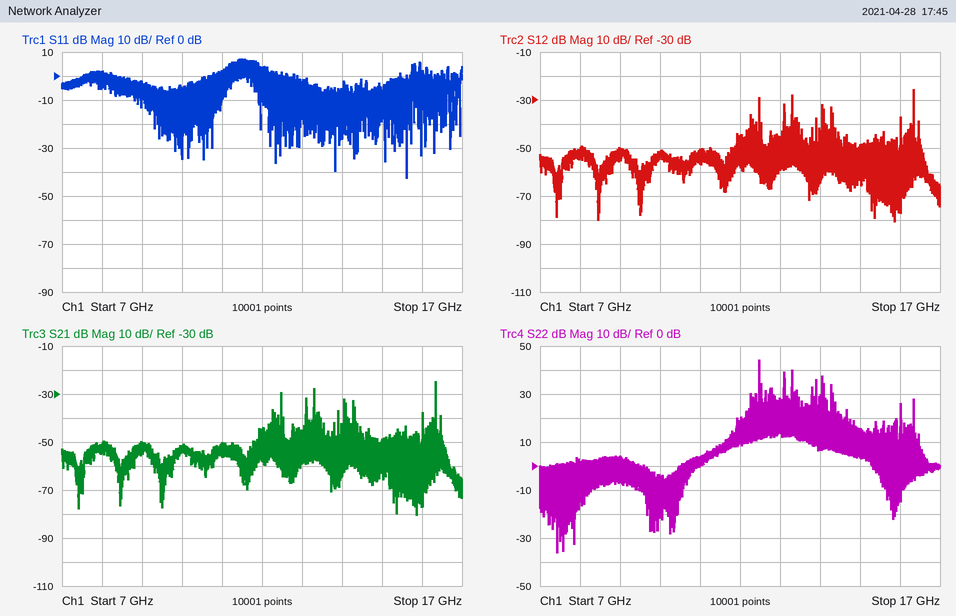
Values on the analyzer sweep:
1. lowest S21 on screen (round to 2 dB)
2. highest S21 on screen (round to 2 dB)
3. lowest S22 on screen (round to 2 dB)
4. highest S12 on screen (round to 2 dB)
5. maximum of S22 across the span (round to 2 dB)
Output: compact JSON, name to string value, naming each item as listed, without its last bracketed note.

{"lowest S21 on screen": "-80 dB", "highest S21 on screen": "-24 dB", "lowest S22 on screen": "-36 dB", "highest S12 on screen": "-26 dB", "maximum of S22 across the span": "44 dB"}
